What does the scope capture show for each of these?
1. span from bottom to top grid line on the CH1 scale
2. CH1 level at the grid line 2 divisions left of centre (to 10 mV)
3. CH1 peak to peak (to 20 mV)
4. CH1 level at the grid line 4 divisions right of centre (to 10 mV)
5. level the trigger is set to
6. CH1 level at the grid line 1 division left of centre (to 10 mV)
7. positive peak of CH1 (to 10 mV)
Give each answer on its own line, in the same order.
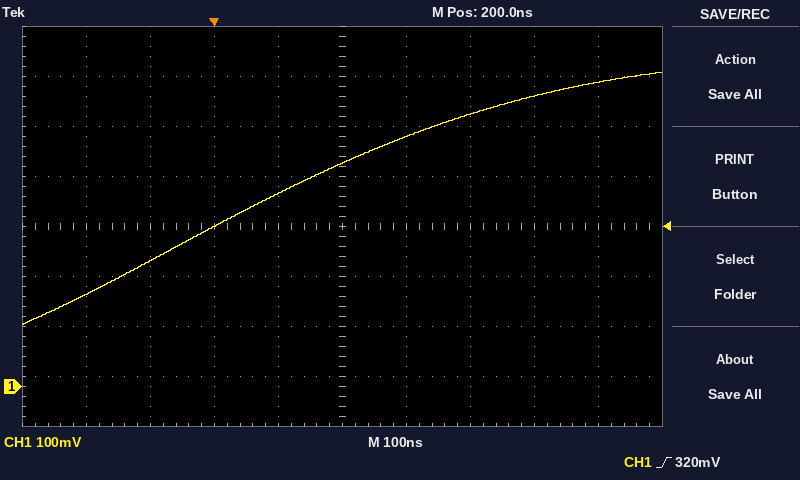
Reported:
800 mV
320 mV
500 mV
610 mV
320 mV
390 mV
630 mV
